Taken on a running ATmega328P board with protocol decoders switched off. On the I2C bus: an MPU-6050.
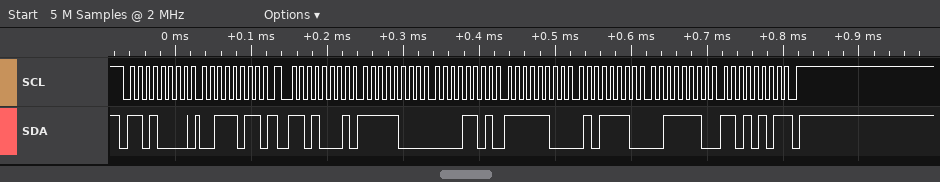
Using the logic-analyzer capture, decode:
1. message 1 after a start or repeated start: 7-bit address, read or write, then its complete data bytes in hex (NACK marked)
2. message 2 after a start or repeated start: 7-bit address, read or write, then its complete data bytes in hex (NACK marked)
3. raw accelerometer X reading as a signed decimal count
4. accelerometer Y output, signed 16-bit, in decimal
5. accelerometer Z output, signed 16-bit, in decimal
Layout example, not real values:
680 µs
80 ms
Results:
0x68 write: 3B
0x68 read: F8 0D FC 5E 3E D5 NACK
-2035
-930
16085
